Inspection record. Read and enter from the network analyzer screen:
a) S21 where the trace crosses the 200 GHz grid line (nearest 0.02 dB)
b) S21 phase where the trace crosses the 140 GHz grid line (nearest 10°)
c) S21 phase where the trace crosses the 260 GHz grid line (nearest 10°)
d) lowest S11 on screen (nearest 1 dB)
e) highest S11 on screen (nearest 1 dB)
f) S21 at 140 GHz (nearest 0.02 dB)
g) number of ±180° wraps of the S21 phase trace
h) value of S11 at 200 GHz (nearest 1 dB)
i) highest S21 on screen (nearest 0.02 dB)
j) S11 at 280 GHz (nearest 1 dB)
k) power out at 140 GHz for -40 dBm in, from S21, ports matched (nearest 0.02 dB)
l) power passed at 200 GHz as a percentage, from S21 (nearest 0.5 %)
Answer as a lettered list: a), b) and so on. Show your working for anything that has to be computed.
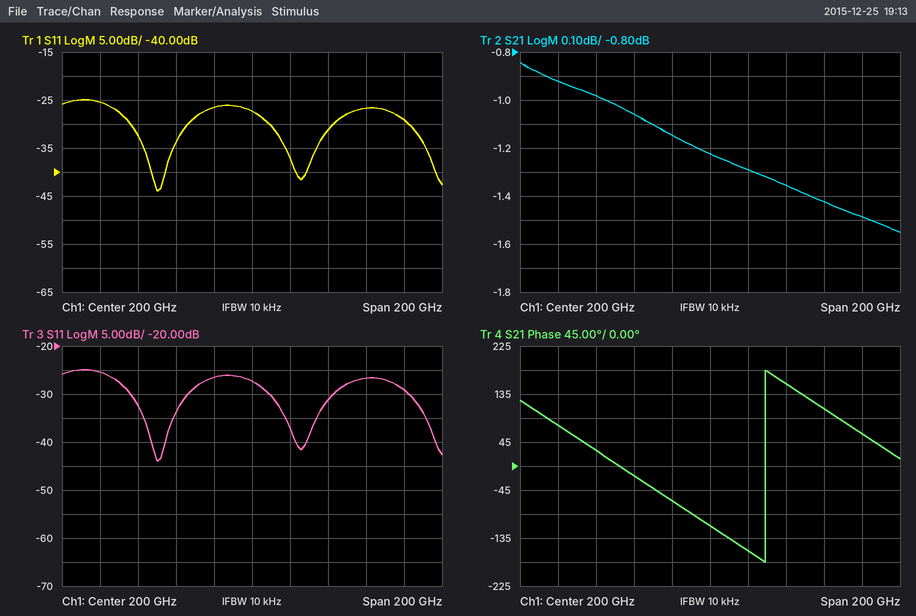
a) -1.22 dB
b) 30°
c) 110°
d) -44 dB
e) -25 dB
f) -0.98 dB
g) 1
h) -27 dB
i) -0.84 dB
j) -29 dB
k) -40 dBm + (-0.98 dB) = -40.98 dBm
l) 10^(-1.22/10) ≈ 75.5 %
